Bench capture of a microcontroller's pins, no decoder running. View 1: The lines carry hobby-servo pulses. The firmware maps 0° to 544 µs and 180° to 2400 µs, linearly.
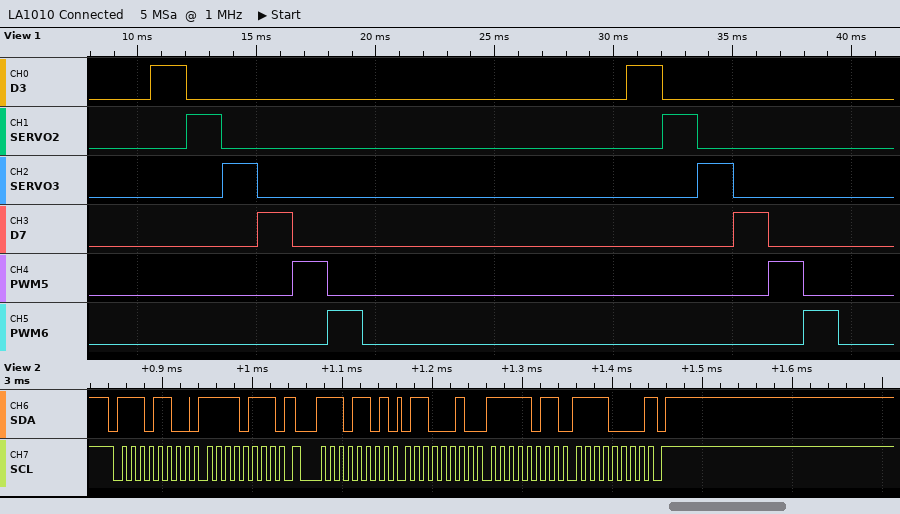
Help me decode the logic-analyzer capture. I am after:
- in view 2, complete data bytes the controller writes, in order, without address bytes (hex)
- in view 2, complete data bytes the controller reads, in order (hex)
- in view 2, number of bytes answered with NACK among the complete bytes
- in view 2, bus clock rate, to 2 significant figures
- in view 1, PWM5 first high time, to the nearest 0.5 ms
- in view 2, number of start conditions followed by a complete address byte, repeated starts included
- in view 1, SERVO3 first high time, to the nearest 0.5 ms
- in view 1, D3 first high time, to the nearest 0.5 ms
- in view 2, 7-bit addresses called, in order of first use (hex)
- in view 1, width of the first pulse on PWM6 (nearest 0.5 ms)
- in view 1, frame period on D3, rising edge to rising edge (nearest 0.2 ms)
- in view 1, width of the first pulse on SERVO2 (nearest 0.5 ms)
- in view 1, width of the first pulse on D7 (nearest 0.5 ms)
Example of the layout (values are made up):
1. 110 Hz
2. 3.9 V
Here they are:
1. F7
2. 62 FB F0
3. 1
4. 100 kHz
5. 1.5 ms
6. 2
7. 1.5 ms
8. 1.5 ms
9. 0x76
10. 1.5 ms
11. 20.0 ms
12. 1.5 ms
13. 1.5 ms
